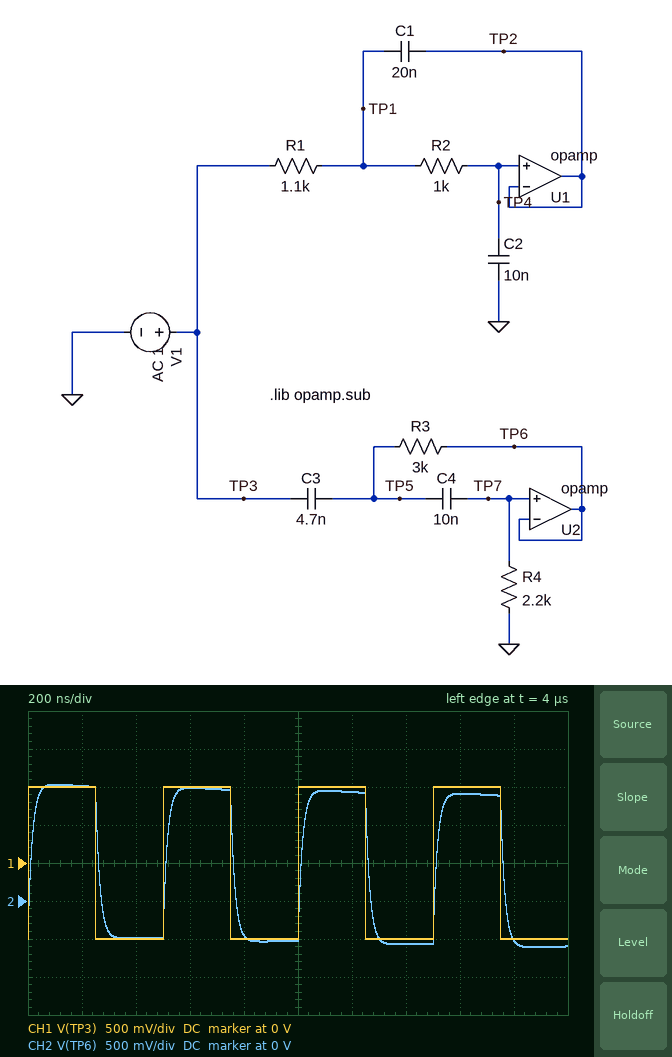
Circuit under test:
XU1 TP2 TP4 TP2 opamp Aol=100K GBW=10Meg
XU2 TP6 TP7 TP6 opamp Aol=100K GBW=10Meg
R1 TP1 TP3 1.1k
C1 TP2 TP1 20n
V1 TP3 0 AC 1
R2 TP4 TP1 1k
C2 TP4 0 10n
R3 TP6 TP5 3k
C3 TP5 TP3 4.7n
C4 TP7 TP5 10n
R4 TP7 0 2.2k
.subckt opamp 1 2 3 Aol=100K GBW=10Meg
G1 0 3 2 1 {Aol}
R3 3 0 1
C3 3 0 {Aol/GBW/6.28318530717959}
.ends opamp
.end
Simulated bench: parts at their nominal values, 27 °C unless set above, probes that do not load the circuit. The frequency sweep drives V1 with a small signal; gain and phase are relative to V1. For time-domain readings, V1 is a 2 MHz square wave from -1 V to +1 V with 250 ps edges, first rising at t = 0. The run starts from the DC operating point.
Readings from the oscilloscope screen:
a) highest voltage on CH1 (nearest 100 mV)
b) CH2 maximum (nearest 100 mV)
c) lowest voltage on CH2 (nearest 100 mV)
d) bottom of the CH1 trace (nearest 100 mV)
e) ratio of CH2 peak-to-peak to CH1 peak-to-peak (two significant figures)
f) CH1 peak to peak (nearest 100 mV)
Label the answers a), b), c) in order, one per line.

a) 1.0 V
b) 1.5 V
c) -600 mV
d) -1.0 V
e) 1.1
f) 2.0 V
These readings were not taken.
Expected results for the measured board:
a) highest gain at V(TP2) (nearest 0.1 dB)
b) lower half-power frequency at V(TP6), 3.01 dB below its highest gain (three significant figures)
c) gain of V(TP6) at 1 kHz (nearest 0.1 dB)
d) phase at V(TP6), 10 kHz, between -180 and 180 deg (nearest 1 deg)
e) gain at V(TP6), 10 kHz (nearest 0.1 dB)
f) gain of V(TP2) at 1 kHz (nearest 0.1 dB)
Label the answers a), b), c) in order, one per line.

a) 0 dB
b) 19.1 kHz
c) -38.5 dB
d) 85 deg
e) -7.1 dB
f) 0 dB
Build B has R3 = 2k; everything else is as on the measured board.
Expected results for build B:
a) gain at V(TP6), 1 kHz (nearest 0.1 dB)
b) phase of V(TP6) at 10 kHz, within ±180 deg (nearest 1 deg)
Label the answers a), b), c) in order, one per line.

a) -41.8 dB
b) 96 deg
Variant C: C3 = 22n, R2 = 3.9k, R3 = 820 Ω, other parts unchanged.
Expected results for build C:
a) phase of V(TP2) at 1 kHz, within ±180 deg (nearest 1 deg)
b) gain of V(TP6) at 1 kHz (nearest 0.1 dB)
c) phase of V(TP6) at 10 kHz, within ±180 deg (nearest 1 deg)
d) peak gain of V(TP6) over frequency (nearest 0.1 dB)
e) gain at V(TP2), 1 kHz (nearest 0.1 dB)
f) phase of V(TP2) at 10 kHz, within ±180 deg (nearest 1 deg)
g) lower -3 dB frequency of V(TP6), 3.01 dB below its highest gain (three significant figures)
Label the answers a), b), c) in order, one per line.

a) -18 deg
b) -36.1 dB
c) 71 deg
d) 0.1 dB
e) -0.1 dB
f) -127 deg
g) 7.53 kHz
